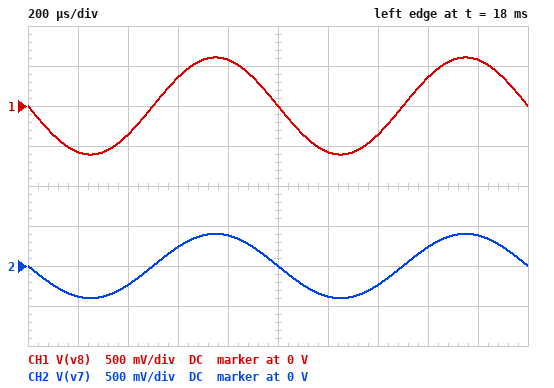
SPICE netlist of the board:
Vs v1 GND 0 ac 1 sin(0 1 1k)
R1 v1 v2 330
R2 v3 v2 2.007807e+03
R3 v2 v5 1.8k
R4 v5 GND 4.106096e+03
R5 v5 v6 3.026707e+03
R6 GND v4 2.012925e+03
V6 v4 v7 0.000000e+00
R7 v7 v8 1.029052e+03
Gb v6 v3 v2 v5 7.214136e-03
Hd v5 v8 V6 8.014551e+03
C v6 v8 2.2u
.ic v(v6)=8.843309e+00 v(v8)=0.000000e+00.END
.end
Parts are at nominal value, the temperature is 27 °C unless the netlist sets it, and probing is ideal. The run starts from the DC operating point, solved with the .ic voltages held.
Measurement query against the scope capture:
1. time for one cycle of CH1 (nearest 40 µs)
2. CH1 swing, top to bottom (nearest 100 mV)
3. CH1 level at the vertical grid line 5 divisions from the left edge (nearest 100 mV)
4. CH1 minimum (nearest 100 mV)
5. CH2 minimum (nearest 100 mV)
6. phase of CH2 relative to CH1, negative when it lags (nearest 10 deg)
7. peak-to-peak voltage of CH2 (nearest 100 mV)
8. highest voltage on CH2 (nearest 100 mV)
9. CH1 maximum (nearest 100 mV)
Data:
1.00 ms
1.2 V
0 V
-600 mV
-400 mV
0 deg
800 mV
400 mV
600 mV
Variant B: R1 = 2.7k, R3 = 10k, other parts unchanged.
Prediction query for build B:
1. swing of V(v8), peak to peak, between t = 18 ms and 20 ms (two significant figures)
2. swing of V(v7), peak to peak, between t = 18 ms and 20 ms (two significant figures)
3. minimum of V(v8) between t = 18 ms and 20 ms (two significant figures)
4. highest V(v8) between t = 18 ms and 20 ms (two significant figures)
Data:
1.1 V
730 mV
-550 mV
550 mV
